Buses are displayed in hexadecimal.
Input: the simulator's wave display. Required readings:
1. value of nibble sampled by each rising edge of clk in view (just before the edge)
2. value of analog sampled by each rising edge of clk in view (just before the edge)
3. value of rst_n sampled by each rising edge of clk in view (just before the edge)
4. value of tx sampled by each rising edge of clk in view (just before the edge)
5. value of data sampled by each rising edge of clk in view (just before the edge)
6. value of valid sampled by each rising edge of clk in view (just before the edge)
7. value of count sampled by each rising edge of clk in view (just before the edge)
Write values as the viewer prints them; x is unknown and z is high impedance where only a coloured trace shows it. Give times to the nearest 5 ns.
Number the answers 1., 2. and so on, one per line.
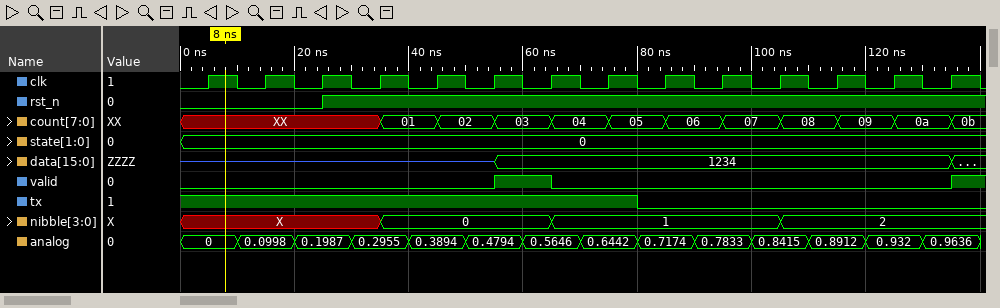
1. X, X, X, X, 0, 0, 0, 1, 1, 1, 1, 2, 2, 2
2. 0, 0.0998, 0.1987, 0.2955, 0.3894, 0.4794, 0.5646, 0.6442, 0.7174, 0.7833, 0.8415, 0.8912, 0.932, 0.9636
3. 0 0 0 1 1 1 1 1 1 1 1 1 1 1
4. 1 1 1 1 1 1 1 1 0 0 0 0 0 0
5. z, z, z, z, z, z, 1234, 1234, 1234, 1234, 1234, 1234, 1234, 1234
6. 0 0 0 0 0 0 1 0 0 0 0 0 0 0
7. XX, XX, XX, XX, 01, 02, 03, 04, 05, 06, 07, 08, 09, 0a
